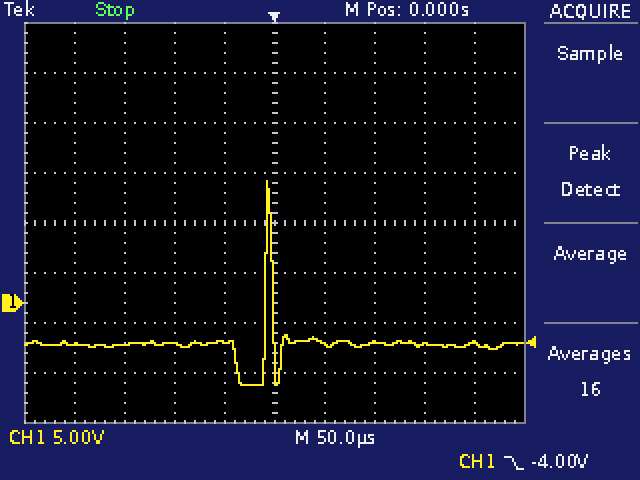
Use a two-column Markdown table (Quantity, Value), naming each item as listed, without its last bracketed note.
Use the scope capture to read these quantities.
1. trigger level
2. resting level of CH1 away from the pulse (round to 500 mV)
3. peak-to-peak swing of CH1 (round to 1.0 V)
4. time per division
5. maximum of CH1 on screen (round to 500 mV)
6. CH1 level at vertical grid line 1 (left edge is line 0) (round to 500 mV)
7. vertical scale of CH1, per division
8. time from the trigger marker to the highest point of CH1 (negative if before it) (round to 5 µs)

| Quantity | Value |
|---|---|
| trigger level | -4.00 V |
| resting level of CH1 away from the pulse | -4.0 V |
| peak-to-peak swing of CH1 | 20.0 V |
| time per division | 50 µs |
| maximum of CH1 on screen | 12.0 V |
| CH1 level at vertical grid line 1 (left edge is line 0) | -4.0 V |
| vertical scale of CH1, per division | 5 V |
| time from the trigger marker to the highest point of CH1 (negative if before it) | -5 µs |
